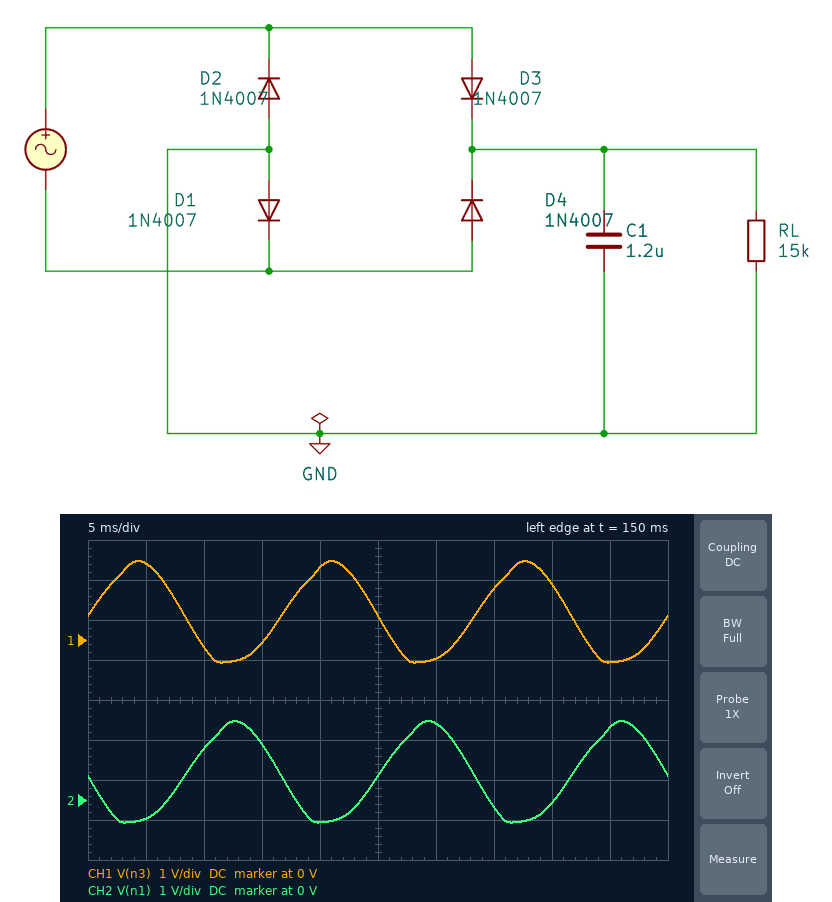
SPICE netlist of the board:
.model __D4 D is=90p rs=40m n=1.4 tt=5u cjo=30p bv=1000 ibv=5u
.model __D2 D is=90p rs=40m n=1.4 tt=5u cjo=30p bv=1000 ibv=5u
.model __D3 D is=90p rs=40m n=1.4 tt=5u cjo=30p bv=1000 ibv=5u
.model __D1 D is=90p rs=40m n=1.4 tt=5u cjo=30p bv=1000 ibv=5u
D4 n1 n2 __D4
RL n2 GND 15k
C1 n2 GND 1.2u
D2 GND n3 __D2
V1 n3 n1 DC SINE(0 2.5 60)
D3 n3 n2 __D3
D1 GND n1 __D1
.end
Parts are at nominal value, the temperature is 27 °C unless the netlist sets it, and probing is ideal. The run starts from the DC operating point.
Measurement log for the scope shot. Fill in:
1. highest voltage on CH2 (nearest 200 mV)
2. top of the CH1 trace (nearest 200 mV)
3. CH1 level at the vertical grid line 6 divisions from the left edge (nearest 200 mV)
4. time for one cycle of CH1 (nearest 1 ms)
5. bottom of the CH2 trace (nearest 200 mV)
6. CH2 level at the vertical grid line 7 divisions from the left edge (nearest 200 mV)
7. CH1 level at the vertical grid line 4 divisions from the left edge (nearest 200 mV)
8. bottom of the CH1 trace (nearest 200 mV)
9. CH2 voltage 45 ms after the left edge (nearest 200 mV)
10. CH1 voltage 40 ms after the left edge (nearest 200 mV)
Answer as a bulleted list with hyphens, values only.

- 2.0 V
- 2.0 V
- -400 mV
- 17 ms
- -600 mV
- -200 mV
- 1.8 V
- -600 mV
- 1.8 V
- 1.4 V
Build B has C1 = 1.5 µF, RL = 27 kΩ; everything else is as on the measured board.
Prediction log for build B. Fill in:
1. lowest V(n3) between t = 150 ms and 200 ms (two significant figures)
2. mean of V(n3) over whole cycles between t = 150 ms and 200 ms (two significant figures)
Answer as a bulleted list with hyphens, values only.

- -550 mV
- 680 mV
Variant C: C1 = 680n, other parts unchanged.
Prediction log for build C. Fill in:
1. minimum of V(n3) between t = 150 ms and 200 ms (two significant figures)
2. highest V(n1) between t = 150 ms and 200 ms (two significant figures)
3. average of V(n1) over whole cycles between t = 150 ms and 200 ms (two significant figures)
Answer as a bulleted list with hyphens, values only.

- -550 mV
- 2.0 V
- 590 mV
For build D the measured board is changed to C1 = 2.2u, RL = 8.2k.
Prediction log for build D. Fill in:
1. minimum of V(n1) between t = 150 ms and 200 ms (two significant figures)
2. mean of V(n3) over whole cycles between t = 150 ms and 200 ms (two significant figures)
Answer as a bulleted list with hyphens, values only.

- -580 mV
- 610 mV
